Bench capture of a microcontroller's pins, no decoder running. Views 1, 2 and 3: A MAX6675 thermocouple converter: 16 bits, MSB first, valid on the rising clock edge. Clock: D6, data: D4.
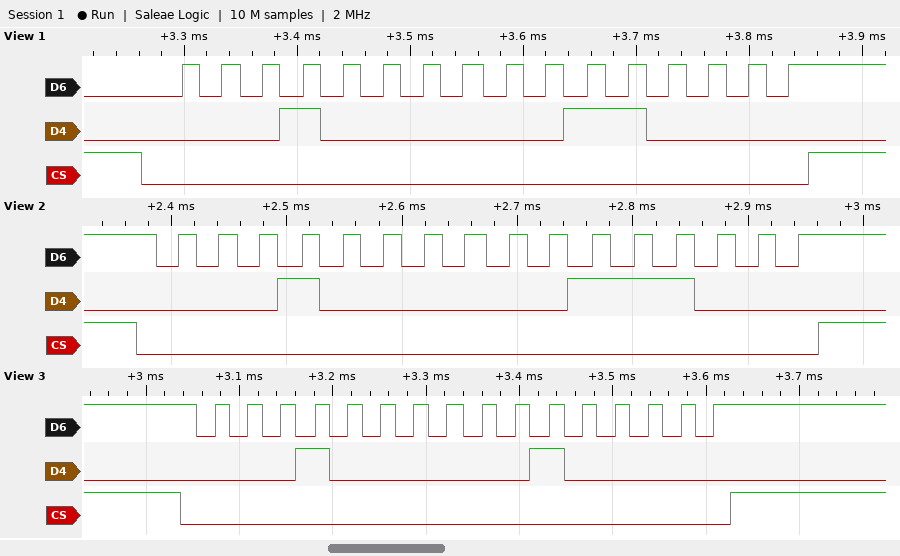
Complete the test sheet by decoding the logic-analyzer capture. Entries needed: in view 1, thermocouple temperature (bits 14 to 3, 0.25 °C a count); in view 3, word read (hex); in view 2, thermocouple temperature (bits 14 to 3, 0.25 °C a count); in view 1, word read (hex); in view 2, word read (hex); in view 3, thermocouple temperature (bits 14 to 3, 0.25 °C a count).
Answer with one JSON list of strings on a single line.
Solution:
["129.50 °C", "0x1020", "129.75 °C", "0x1030", "0x1038", "129.00 °C"]
